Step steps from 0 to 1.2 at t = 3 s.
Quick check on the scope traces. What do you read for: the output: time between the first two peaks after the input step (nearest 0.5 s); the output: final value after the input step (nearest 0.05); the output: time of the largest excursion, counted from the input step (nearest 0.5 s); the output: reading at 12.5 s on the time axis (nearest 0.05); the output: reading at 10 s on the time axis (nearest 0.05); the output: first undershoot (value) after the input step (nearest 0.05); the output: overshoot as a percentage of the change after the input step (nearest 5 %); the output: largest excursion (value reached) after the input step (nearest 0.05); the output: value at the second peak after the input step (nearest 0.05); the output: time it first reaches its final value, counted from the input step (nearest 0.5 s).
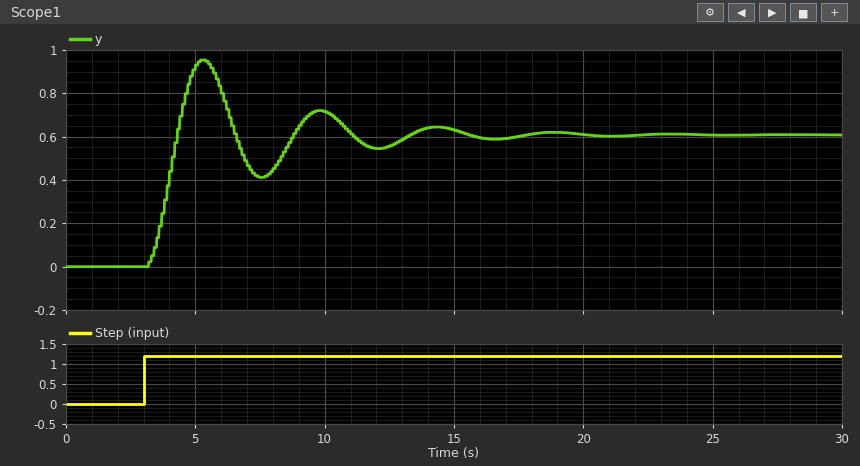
4.5 s
0.60
2.5 s
0.55
0.70
0.40
55 %
0.95
0.70
1.5 s
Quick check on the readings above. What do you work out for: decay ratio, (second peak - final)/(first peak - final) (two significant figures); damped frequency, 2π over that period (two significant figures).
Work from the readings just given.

0.29
1.4 rad/s
